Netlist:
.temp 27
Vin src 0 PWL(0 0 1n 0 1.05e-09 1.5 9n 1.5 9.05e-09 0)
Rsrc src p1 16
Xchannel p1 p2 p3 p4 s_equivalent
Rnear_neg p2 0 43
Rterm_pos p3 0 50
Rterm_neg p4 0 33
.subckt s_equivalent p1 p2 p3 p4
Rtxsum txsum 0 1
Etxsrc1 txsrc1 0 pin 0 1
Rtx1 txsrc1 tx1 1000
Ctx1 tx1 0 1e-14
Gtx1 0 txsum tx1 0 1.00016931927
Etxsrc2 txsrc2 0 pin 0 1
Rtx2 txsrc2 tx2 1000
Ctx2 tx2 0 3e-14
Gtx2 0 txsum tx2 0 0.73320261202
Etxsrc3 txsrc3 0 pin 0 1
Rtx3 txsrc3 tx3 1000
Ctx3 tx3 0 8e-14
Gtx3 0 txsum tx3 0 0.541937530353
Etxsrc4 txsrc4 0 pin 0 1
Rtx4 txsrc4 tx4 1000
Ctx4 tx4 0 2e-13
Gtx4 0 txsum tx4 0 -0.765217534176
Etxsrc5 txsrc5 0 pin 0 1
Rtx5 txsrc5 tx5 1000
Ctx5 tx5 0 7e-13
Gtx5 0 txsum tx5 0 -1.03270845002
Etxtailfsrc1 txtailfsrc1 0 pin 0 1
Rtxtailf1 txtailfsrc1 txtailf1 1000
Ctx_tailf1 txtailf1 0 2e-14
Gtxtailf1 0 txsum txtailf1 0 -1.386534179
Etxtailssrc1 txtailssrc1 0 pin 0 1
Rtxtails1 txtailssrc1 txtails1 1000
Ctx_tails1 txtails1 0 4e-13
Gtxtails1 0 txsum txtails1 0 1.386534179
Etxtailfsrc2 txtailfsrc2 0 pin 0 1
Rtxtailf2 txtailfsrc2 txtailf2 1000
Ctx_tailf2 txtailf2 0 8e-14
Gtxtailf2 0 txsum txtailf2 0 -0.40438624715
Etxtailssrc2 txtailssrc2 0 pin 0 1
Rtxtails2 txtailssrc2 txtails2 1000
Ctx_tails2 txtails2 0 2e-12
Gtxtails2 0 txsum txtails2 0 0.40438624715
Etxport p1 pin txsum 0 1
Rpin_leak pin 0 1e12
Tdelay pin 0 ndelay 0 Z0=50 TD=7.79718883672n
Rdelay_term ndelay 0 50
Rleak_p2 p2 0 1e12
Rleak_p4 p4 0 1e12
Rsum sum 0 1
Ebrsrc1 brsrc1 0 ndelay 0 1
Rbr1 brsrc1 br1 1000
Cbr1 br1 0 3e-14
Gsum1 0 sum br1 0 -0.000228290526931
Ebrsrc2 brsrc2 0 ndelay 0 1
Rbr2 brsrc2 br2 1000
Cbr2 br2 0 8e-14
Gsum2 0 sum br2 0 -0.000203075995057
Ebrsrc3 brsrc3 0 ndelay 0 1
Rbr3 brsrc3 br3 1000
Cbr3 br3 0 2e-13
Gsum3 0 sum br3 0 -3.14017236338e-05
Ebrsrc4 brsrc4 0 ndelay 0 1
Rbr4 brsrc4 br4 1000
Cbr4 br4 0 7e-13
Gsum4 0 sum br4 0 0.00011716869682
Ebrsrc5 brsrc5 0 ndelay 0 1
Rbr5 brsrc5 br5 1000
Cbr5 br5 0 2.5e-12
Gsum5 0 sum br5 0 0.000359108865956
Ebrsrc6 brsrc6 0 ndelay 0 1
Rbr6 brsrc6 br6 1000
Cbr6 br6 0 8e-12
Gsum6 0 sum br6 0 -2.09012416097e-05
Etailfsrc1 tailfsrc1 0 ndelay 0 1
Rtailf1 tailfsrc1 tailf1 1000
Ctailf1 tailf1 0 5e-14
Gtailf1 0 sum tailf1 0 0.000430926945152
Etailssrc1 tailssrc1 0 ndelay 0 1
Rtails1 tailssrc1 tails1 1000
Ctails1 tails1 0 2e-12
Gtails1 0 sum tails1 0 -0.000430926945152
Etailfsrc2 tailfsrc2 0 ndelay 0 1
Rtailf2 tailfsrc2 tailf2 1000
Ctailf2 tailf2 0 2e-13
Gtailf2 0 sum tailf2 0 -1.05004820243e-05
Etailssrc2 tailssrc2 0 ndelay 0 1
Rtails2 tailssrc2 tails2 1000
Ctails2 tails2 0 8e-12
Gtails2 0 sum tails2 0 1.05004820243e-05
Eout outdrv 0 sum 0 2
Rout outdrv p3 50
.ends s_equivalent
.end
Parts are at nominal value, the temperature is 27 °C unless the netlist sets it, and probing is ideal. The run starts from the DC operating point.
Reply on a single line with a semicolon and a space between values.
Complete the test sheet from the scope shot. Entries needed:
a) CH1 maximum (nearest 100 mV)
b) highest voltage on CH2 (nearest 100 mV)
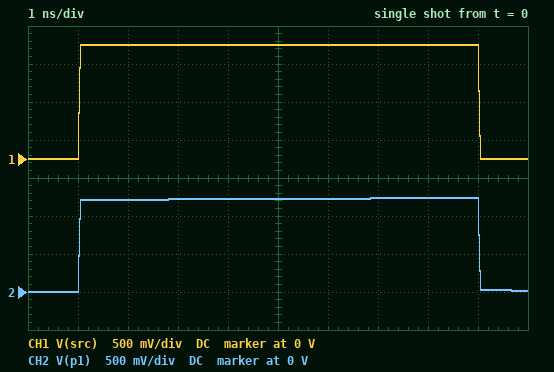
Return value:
1.5 V; 1.2 V
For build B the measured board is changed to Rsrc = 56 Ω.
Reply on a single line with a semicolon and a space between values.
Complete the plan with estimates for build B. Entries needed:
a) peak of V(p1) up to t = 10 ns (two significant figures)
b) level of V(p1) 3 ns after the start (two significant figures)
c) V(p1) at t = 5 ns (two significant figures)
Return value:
850 mV; 830 mV; 840 mV
